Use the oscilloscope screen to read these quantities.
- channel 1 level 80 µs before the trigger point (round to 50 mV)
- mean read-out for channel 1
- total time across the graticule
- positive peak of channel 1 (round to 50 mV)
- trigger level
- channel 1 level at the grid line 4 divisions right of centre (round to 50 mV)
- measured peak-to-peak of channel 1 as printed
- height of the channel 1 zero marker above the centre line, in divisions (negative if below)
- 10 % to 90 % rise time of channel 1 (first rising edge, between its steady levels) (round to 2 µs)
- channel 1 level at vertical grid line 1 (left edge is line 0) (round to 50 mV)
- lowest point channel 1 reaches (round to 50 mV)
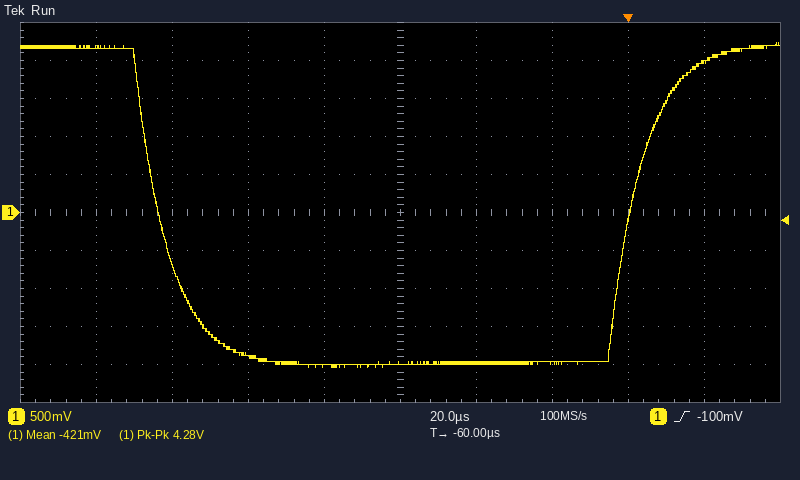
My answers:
-2.00 V
-421 mV
200 µs
2.25 V
-100 mV
2.00 V
4.28 V
0.0 div
18 µs
2.20 V
-2.05 V
